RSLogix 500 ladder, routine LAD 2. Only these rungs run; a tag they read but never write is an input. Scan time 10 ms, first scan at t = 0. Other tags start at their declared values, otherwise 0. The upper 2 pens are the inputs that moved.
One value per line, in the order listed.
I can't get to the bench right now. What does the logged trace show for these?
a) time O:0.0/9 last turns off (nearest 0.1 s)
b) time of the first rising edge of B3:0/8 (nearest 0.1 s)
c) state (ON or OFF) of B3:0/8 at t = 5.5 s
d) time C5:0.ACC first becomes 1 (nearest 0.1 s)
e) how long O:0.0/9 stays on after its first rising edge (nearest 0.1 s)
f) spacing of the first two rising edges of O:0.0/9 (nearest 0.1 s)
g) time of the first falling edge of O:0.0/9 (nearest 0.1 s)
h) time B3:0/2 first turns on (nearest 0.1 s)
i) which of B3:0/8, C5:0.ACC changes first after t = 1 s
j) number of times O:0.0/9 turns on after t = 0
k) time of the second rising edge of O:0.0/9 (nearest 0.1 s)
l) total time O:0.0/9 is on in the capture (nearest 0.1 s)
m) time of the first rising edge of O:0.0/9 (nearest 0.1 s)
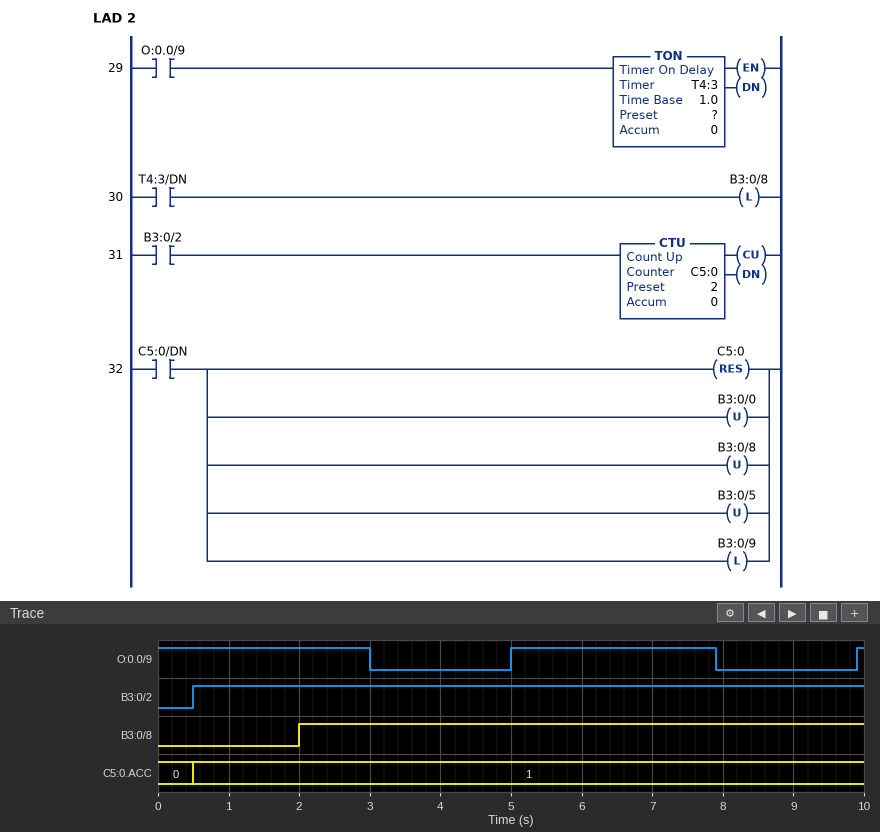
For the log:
7.9 s
2.0 s
ON
0.5 s
2.9 s
4.9 s
3.0 s
0.5 s
B3:0/8
2
9.9 s
6.0 s
5.0 s
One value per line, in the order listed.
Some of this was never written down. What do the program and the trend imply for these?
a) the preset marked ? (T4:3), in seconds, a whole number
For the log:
2 s
